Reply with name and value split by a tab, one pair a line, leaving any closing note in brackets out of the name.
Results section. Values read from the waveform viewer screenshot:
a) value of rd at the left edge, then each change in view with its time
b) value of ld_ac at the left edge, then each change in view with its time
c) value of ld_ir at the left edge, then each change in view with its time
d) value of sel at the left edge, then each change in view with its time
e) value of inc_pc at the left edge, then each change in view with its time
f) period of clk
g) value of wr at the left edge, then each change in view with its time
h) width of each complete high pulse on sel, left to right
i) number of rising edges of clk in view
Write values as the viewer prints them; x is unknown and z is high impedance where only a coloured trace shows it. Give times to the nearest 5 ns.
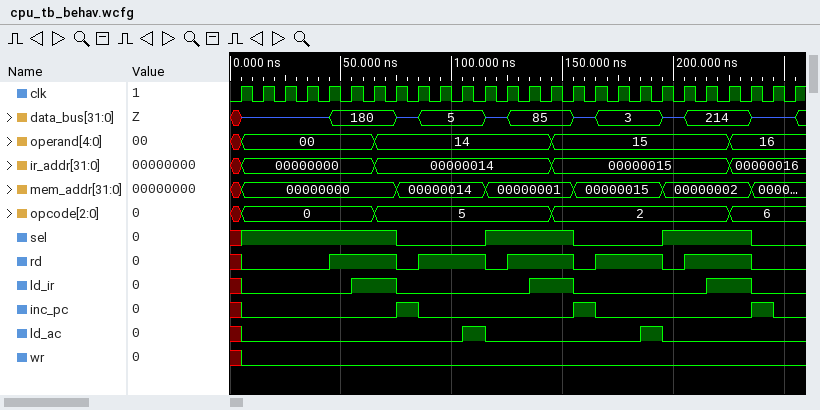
value of rd at the left edge, then each change in view with its time	x, 0 at 5 ns, 1 at 45 ns, 0 at 75 ns, 1 at 85 ns, 0 at 115 ns, 1 at 125 ns, 0 at 155 ns, 1 at 165 ns, 0 at 195 ns, 1 at 205 ns, 0 at 235 ns
value of ld_ac at the left edge, then each change in view with its time	x, 0 at 5 ns, 1 at 105 ns, 0 at 115 ns, 1 at 185 ns, 0 at 195 ns
value of ld_ir at the left edge, then each change in view with its time	x, 0 at 5 ns, 1 at 55 ns, 0 at 75 ns, 1 at 135 ns, 0 at 155 ns, 1 at 215 ns, 0 at 235 ns
value of sel at the left edge, then each change in view with its time	x, 1 at 5 ns, 0 at 75 ns, 1 at 115 ns, 0 at 155 ns, 1 at 195 ns, 0 at 235 ns
value of inc_pc at the left edge, then each change in view with its time	x, 0 at 5 ns, 1 at 75 ns, 0 at 85 ns, 1 at 155 ns, 0 at 165 ns, 1 at 235 ns, 0 at 245 ns
period of clk	10 ns
value of wr at the left edge, then each change in view with its time	x, 0 at 5 ns
width of each complete high pulse on sel, left to right	40 ns, 40 ns
number of rising edges of clk in view	26
